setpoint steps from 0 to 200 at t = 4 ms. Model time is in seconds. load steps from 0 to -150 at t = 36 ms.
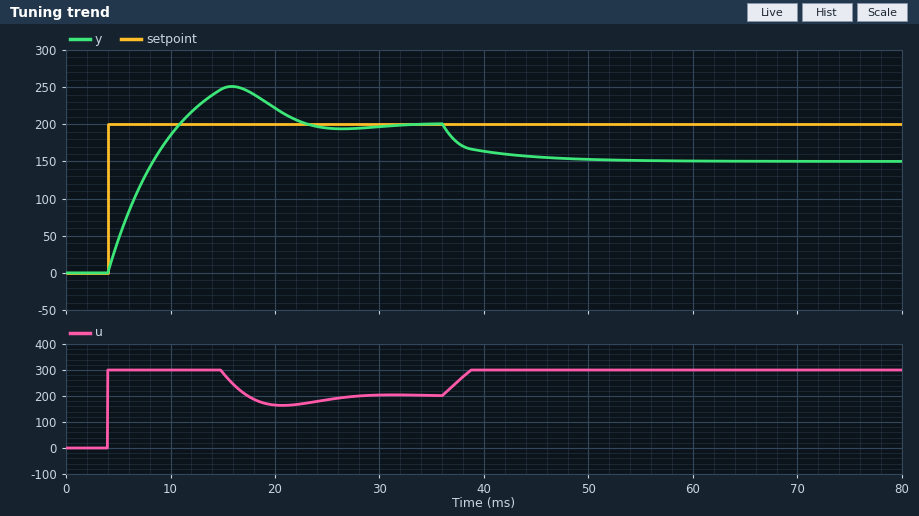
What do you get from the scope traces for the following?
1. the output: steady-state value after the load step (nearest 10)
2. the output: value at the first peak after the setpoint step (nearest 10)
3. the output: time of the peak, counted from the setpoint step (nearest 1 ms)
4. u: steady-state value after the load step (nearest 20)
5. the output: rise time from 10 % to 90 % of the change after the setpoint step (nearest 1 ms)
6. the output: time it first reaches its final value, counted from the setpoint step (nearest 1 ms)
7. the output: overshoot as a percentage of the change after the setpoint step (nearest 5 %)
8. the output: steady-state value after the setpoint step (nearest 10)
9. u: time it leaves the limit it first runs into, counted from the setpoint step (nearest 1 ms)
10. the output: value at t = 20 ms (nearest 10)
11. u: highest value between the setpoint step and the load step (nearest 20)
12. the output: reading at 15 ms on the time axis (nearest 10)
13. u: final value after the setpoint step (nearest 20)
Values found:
150
250
12 ms
300
5 ms
7 ms
25 %
200
11 ms
220
300
250
200
